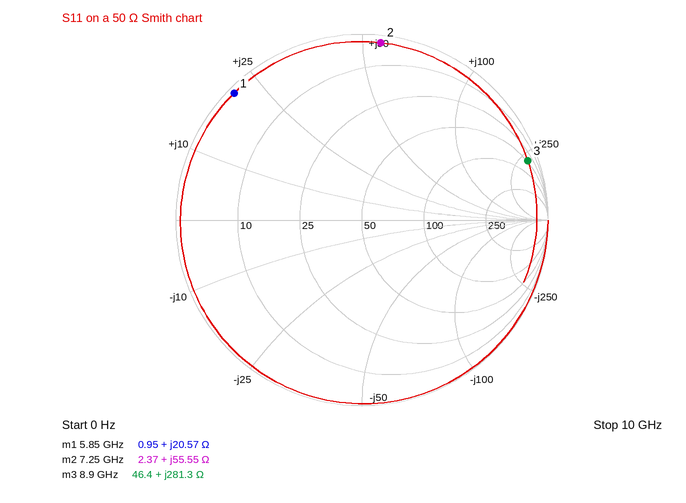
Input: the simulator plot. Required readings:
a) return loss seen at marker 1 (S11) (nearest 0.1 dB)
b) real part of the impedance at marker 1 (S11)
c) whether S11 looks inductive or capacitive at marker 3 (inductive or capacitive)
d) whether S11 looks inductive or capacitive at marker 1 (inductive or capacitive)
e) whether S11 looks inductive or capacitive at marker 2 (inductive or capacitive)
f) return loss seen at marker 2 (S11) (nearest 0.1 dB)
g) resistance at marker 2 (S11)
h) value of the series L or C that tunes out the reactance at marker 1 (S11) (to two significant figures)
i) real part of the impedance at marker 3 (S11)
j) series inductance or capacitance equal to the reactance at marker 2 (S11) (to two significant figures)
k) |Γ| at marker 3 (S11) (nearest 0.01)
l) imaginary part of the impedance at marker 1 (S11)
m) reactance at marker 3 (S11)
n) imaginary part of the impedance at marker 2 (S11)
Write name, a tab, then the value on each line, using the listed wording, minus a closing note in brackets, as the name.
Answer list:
return loss seen at marker 1 (S11)	0.3 dB
real part of the impedance at marker 1	0.95 Ω
whether S11 looks inductive or capacitive at marker 3	inductive
whether S11 looks inductive or capacitive at marker 1	inductive
whether S11 looks inductive or capacitive at marker 2	inductive
return loss seen at marker 2 (S11)	0.4 dB
resistance at marker 2	2.37 Ω
value of the series L or C that tunes out the reactance at marker 1 (S11)	1.3 pF
real part of the impedance at marker 3	46.4 Ω
series inductance or capacitance equal to the reactance at marker 2 (S11)	1.2 nH
|Γ| at marker 3 (S11)	0.95
imaginary part of the impedance at marker 1	+20.57 Ω
reactance at marker 3	+281.3 Ω
imaginary part of the impedance at marker 2	+55.55 Ω
